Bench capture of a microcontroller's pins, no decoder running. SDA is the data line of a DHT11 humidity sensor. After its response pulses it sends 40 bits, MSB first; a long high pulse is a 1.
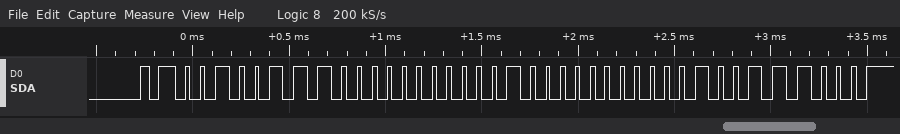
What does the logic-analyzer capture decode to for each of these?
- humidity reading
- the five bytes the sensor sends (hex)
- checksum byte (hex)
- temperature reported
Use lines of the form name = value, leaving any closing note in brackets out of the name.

humidity reading = 39 %
the five bytes the sensor sends = 27 00 10 01 38
checksum byte = 0x38
temperature reported = 16.1 °C
